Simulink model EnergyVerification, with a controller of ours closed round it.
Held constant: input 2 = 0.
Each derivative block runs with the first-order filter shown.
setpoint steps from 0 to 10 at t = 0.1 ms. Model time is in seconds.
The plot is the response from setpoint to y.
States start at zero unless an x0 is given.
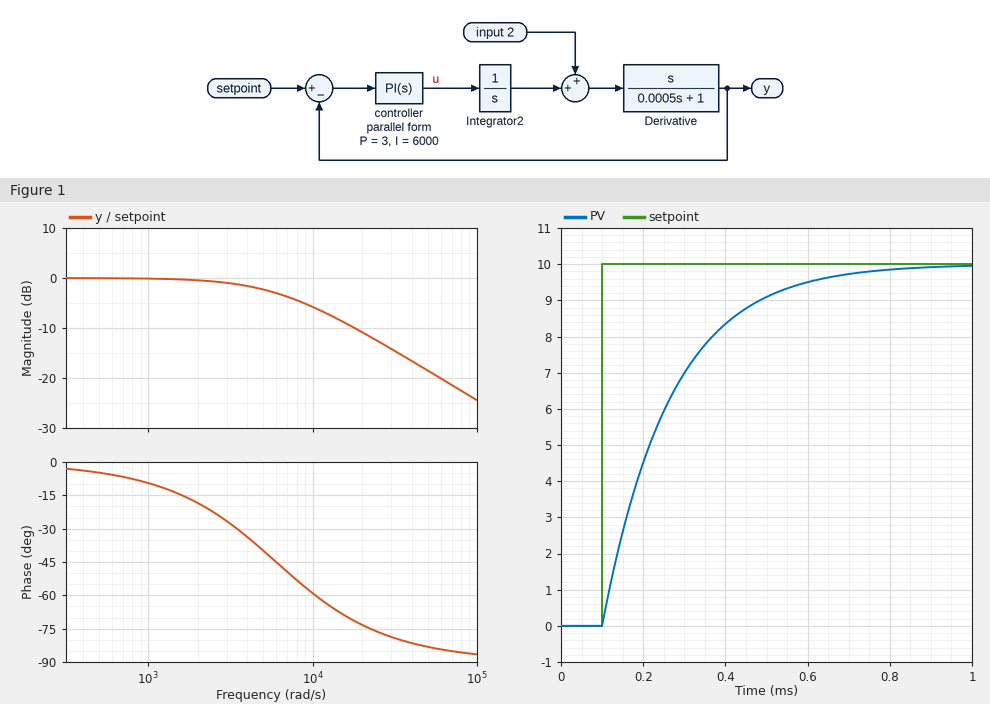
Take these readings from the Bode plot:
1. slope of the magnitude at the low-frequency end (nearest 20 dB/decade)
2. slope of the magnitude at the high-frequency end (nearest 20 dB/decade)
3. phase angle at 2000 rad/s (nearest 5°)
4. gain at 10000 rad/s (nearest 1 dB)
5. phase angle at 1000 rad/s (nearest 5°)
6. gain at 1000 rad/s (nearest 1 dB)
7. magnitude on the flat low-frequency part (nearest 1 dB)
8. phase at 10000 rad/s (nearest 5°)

0 dB/decade
-20 dB/decade
-20°
-6 dB
-10°
0 dB
0 dB
-60°
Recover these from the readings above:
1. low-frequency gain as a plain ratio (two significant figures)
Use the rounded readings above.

1.0
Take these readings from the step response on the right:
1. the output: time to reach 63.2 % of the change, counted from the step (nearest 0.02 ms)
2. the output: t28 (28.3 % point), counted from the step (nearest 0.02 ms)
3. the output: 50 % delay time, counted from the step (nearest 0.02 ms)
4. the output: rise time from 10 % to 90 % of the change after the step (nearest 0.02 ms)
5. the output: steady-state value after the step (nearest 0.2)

0.16 ms
0.06 ms
0.12 ms
0.36 ms
10.0
